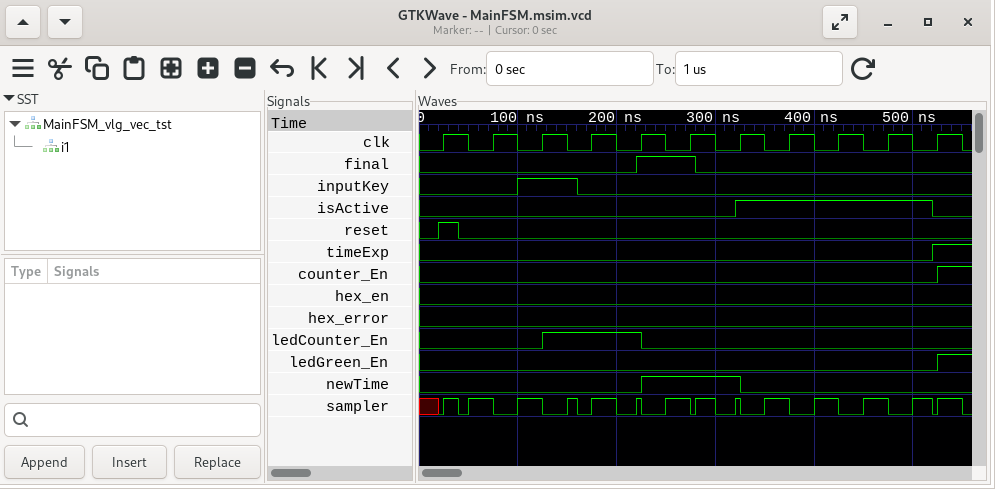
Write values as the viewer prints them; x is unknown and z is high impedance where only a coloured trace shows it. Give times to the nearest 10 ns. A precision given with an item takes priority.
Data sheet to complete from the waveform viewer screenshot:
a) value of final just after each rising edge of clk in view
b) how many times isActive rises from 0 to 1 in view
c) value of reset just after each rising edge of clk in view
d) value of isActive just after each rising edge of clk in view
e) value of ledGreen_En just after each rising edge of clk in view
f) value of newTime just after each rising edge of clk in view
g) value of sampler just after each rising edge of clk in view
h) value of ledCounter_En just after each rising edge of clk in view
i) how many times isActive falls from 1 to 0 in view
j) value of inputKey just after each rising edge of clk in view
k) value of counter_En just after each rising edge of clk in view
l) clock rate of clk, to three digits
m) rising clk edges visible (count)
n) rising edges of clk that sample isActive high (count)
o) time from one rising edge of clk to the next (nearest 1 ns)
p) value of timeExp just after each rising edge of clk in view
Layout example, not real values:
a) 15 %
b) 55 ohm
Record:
a) 0 0 0 0 1 1 0 0 0 0 0
b) 1
c) 1 0 0 0 0 0 0 0 0 0 0
d) 0 0 0 0 0 0 1 1 1 1 0
e) 0 0 0 0 0 0 0 0 0 0 1
f) 0 0 0 0 1 1 0 0 0 0 0
g) 1 0 0 1 0 0 0 0 0 0 1
h) 0 0 1 1 0 0 0 0 0 0 0
i) 1
j) 0 0 1 0 0 0 0 0 0 0 0
k) 0 0 0 0 0 0 0 0 0 0 1
l) 20.0 MHz
m) 11
n) 4
o) 50 ns
p) 0 0 0 0 0 0 0 0 0 0 1
